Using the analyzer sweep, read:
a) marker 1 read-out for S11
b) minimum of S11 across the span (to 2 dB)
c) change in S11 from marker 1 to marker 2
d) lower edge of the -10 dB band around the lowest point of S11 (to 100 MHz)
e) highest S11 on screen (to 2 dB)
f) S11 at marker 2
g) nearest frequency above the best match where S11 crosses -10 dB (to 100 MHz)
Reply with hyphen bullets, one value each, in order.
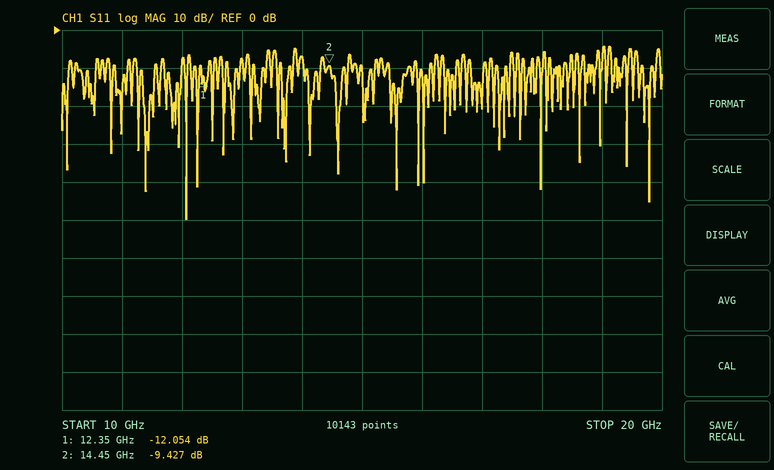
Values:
- -12.054 dB
- -50 dB
- 2.627 dB
- 12.0 GHz
- -4 dB
- -9.427 dB
- 12.1 GHz
